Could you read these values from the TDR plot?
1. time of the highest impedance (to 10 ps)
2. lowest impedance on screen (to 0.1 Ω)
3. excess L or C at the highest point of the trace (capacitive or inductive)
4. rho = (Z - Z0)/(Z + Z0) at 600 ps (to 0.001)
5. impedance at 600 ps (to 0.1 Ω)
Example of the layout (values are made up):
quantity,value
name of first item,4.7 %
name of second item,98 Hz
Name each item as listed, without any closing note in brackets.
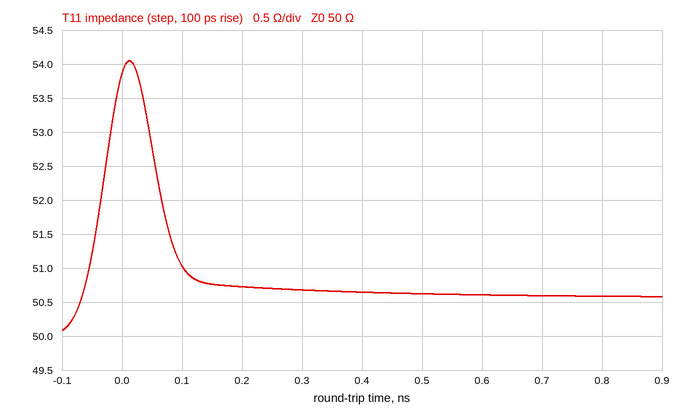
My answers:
quantity,value
time of the highest impedance,10 ps
lowest impedance on screen,50.1 Ω
excess L or C at the highest point of the trace,inductive
rho = (Z - Z0)/(Z + Z0) at 600 ps,+0.006
impedance at 600 ps,50.6 Ω
